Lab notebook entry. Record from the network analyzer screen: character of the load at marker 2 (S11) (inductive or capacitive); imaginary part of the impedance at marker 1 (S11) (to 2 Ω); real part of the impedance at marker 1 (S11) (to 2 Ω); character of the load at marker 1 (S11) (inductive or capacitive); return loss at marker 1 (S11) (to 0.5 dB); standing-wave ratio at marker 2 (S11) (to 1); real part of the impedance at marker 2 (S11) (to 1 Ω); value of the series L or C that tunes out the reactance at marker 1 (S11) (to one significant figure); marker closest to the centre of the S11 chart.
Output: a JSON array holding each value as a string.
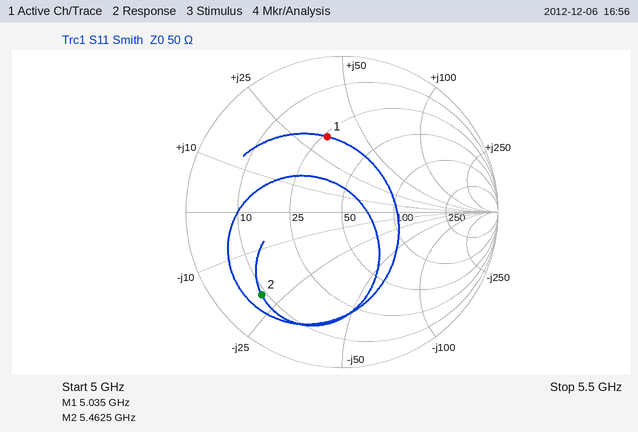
["capacitive", "+34 Ω", "26 Ω", "inductive", "6.0 dB", "7", "9 Ω", "900 fF", "marker 1"]
